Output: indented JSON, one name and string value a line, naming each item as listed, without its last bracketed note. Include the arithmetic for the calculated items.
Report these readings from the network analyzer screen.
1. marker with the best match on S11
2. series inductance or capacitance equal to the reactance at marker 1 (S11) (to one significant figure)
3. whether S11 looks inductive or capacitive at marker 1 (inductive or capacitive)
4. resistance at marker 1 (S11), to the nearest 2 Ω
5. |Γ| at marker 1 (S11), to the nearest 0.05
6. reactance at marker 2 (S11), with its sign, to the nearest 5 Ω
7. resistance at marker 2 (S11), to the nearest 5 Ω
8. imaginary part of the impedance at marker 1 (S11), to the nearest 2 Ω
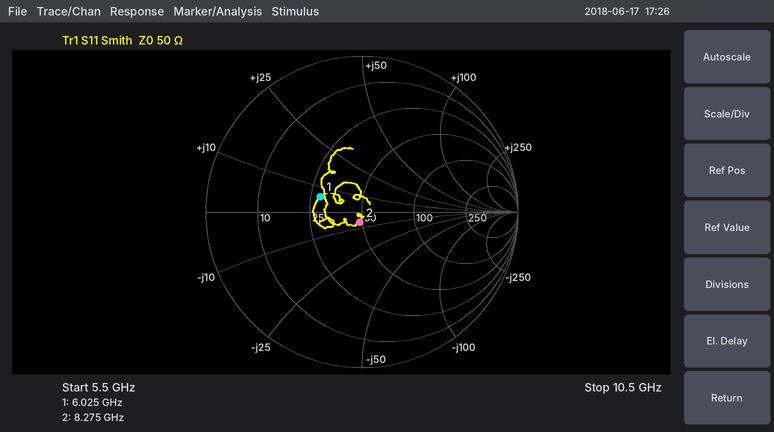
{
  "marker with the best match on S11": "marker 2",
  "series inductance or capacitance equal to the reactance at marker 1 (S11)": "L = 6 Ω/(2π × 6.025 GHz) ≈ 158 pH, so 200 pH to one significant figure",
  "whether S11 looks inductive or capacitive at marker 1": "inductive",
  "resistance at marker 1 (S11), to the nearest 2 Ω": "28 Ω",
  "|Γ| at marker 1 (S11), to the nearest 0.05": "0.30",
  "reactance at marker 2 (S11), with its sign, to the nearest 5 Ω": "-5 Ω",
  "resistance at marker 2 (S11), to the nearest 5 Ω": "50 Ω",
  "imaginary part of the impedance at marker 1 (S11), to the nearest 2 Ω": "+6 Ω"
}
